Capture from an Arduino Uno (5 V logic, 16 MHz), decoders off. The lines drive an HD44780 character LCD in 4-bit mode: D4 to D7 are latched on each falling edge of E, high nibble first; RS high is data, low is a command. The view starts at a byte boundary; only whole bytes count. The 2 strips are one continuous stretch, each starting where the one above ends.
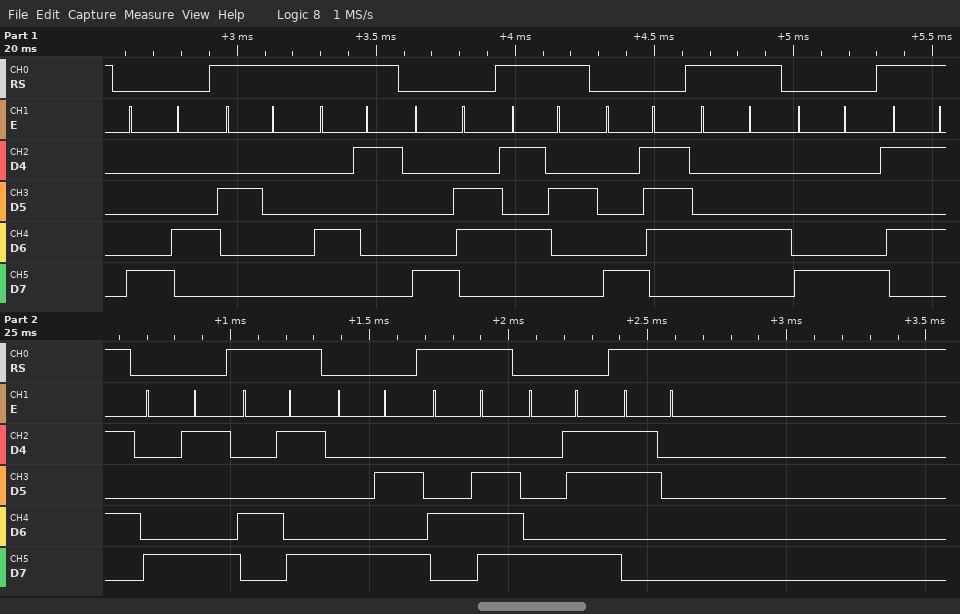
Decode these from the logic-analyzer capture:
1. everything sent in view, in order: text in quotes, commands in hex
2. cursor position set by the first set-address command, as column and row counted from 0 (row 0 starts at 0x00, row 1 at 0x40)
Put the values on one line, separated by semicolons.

0x84 " A" 0x86 "R" 0x87 "D" 0x88 "U" 0x89 "I" 0x8A "N" 0x8B "0"; column 4, row 0
